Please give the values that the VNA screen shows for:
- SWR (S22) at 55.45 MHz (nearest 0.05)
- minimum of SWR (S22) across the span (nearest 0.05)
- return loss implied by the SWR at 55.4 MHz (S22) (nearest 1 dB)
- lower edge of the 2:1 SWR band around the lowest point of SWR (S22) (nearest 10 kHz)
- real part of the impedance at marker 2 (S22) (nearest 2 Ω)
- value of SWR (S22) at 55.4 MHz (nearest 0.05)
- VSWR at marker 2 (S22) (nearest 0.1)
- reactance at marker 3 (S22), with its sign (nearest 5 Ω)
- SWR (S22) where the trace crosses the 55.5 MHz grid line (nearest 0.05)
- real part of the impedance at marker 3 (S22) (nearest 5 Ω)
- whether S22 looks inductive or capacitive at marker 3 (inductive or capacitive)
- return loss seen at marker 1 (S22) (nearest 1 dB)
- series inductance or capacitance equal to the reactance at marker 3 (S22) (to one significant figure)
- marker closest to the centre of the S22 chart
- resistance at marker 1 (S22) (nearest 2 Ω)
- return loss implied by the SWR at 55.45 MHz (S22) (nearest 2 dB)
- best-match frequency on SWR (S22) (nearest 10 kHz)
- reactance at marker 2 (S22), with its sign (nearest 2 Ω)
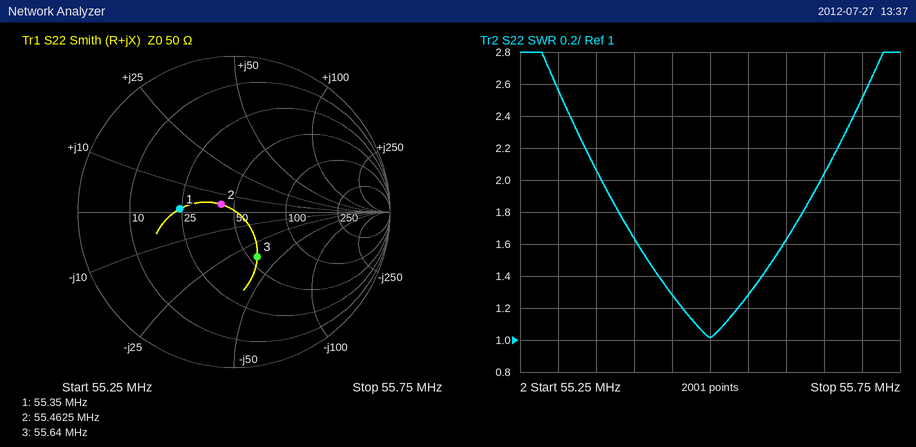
1.30
1.00
12 dB
55.36 MHz
42 Ω
1.65
1.2
-35 Ω
1.00
55 Ω
capacitive
9 dB
80 pF
marker 2
24 Ω
18 dB
55.50 MHz
+4 Ω
